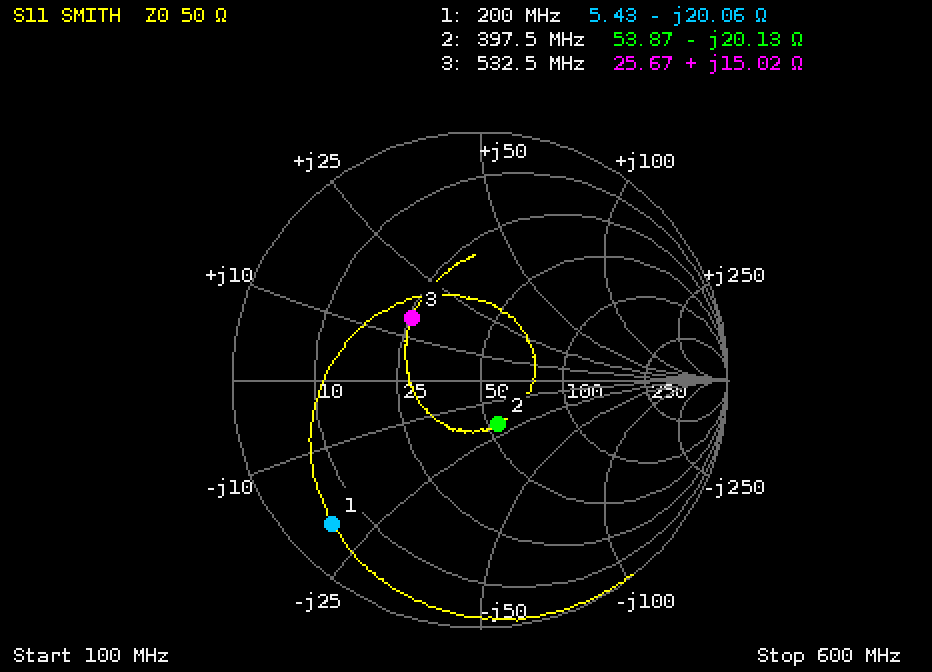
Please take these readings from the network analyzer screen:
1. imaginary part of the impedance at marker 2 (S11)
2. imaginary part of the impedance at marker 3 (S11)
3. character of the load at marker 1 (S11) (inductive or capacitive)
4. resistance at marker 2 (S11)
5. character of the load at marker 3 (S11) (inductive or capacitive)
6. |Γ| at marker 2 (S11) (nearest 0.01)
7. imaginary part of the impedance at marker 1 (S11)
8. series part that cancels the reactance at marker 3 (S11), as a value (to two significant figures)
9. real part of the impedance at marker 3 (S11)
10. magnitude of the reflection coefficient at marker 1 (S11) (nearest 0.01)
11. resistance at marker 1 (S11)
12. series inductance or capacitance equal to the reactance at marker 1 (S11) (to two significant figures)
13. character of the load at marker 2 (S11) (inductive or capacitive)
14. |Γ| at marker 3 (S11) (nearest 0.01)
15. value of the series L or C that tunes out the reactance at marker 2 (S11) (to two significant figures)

-20.13 Ω
+15.02 Ω
capacitive
53.87 Ω
inductive
0.19
-20.06 Ω
20 pF
25.67 Ω
0.83
5.43 Ω
40 pF
capacitive
0.37
8.1 nH
